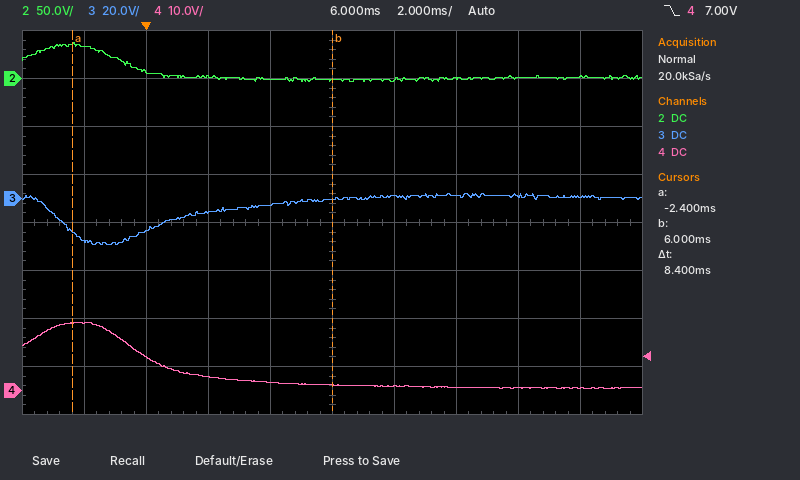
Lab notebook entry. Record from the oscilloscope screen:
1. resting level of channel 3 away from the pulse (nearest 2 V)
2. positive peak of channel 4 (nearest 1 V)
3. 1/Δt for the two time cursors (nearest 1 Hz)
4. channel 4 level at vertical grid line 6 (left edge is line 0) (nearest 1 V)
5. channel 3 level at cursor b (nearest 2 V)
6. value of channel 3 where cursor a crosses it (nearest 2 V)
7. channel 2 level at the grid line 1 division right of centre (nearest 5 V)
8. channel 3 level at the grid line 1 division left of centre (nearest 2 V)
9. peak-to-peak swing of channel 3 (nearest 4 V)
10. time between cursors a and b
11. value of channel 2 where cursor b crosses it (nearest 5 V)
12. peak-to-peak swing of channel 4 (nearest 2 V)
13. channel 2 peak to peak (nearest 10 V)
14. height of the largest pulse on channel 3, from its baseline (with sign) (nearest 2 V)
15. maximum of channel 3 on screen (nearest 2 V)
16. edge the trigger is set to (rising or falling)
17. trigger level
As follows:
0 V
14 V
119 Hz
1 V
0 V
-14 V
0 V
-2 V
20 V
8.4 ms
0 V
14 V
40 V
-20 V
2 V
falling
7.00 V
